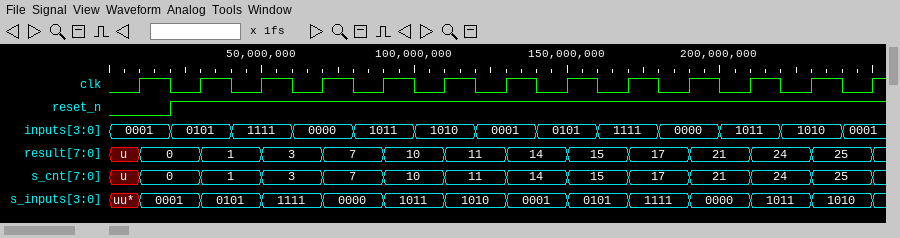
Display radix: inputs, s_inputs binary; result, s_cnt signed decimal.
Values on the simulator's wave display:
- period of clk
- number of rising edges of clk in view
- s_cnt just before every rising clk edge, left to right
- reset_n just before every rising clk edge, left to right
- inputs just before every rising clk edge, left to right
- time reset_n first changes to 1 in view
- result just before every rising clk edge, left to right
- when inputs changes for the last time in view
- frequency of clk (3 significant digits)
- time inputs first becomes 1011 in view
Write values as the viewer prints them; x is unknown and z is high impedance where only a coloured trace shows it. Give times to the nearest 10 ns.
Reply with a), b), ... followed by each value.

a) 20 ns
b) 13
c) u, 0, 1, 3, 7, 10, 11, 14, 15, 17, 21, 24, 25
d) 0 1 1 1 1 1 1 1 1 1 1 1 1
e) 0001, 0101, 1111, 0000, 1011, 1010, 0001, 0101, 1111, 0000, 1011, 1010, 0001
f) 20 ns
g) u, 0, 1, 3, 7, 10, 11, 14, 15, 17, 21, 24, 25
h) 240 ns
i) 50.0 MHz
j) 80 ns
